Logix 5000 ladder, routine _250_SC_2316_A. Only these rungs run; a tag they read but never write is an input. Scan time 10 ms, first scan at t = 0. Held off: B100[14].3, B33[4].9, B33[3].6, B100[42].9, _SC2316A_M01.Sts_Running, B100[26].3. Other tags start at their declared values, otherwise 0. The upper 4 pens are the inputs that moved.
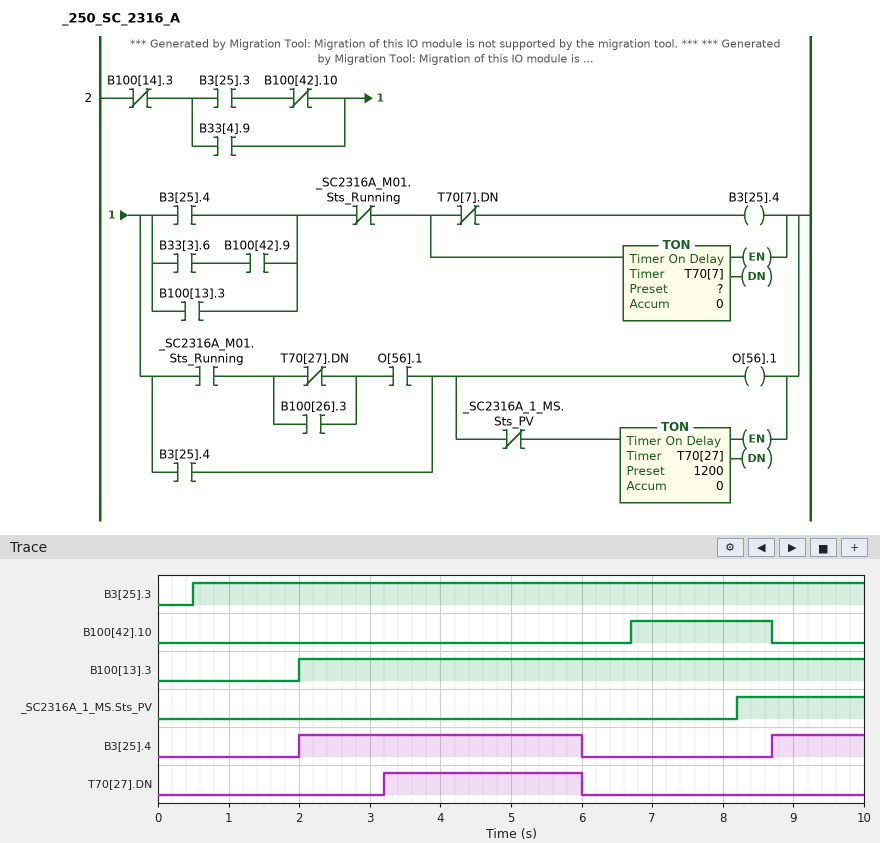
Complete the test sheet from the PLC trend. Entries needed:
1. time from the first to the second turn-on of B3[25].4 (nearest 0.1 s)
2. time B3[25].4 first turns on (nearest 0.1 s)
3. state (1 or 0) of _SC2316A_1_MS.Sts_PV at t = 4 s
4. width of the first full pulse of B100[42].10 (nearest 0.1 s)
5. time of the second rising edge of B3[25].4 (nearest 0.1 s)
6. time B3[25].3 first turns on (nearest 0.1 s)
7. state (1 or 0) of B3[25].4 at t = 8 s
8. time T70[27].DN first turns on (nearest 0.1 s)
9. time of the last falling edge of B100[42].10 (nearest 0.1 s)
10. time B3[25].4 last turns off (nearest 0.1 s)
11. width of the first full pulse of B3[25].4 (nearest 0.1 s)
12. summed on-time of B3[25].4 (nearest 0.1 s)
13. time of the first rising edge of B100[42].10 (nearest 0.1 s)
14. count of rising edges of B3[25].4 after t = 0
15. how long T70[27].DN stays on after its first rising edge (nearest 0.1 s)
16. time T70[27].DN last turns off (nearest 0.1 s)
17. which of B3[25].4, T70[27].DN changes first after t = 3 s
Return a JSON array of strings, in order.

["6.7 s", "2.0 s", "0", "2.0 s", "8.7 s", "0.5 s", "0", "3.2 s", "8.7 s", "6.0 s", "4.0 s", "5.3 s", "6.7 s", "2", "2.8 s", "6.0 s", "T70[27].DN"]
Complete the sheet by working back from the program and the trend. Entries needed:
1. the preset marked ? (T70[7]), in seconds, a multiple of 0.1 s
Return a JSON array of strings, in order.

["4.0 s"]
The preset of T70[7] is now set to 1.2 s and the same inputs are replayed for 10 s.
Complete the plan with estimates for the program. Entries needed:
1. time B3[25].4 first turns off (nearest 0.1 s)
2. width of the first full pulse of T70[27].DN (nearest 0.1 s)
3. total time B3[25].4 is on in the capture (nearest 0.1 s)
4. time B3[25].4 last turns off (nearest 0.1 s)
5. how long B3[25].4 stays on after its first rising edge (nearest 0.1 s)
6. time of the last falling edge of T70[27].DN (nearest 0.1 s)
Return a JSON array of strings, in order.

["3.2 s", "0.0 s", "2.4 s", "9.9 s", "1.2 s", "3.2 s"]
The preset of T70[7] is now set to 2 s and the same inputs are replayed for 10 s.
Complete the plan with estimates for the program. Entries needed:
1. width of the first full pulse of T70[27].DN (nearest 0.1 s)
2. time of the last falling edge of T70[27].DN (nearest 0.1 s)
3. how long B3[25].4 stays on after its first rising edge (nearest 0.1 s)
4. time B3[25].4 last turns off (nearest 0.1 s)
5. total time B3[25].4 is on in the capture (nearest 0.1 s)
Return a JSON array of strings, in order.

["0.8 s", "4.0 s", "2.0 s", "4.0 s", "3.3 s"]
